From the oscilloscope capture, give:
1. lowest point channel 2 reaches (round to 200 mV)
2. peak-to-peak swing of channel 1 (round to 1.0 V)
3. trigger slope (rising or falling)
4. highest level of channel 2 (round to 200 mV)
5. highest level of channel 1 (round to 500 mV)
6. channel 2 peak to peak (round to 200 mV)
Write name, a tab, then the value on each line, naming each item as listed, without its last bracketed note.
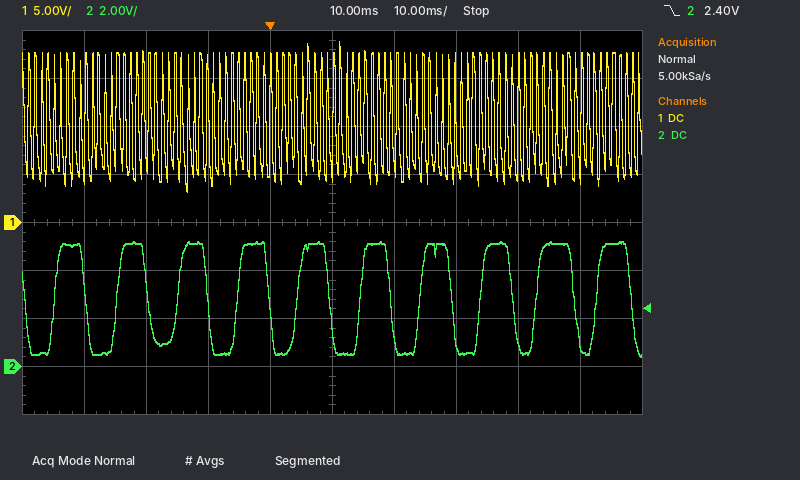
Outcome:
lowest point channel 2 reaches	400 mV
peak-to-peak swing of channel 1	16.0 V
trigger slope	falling
highest level of channel 2	5.2 V
highest level of channel 1	19.0 V
channel 2 peak to peak	4.8 V
